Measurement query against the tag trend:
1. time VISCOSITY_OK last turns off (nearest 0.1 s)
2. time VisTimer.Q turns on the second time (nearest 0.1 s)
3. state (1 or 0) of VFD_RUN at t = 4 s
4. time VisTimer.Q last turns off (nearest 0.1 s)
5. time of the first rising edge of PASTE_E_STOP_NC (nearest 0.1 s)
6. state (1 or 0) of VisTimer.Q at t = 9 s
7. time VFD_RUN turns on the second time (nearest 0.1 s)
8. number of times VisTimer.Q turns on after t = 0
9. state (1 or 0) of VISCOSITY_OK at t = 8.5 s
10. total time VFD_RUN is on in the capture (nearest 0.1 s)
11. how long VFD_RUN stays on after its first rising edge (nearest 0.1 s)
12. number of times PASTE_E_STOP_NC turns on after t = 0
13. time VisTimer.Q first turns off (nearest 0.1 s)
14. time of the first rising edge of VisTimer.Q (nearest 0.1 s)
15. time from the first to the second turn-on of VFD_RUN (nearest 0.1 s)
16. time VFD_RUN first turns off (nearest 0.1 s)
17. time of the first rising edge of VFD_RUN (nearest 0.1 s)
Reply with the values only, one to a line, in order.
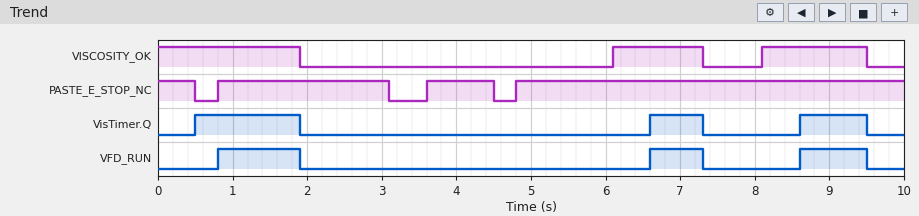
9.5 s
6.6 s
0
9.5 s
0.8 s
1
6.6 s
3
1
2.7 s
1.1 s
3
1.9 s
0.5 s
5.8 s
1.9 s
0.8 s
